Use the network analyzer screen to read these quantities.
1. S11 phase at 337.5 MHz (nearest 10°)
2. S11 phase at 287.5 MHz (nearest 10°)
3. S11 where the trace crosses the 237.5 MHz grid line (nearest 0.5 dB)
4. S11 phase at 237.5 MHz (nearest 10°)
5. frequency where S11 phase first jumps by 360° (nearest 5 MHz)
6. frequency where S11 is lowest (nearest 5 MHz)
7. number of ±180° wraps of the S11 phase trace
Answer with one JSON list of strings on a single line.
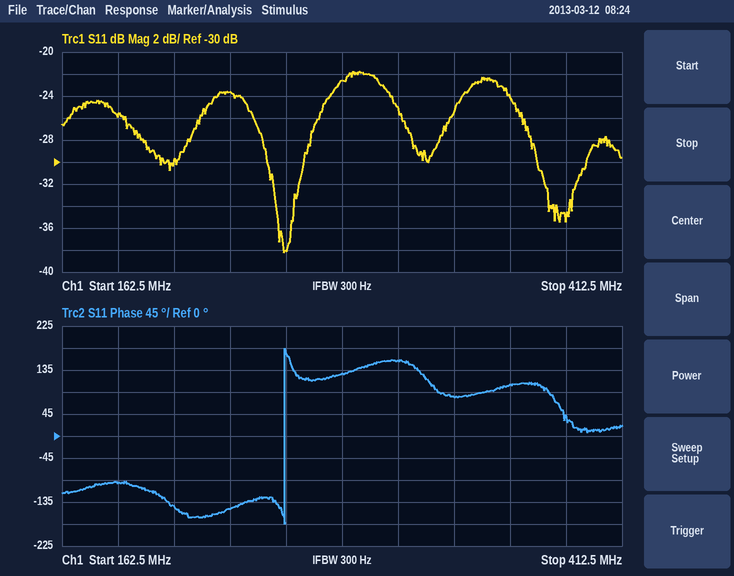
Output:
["80°", "130°", "-23.5 dB", "-150°", "260 MHz", "260 MHz", "1"]
